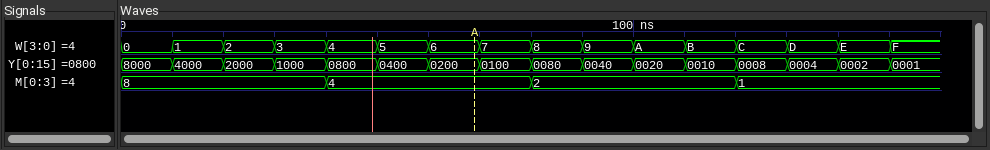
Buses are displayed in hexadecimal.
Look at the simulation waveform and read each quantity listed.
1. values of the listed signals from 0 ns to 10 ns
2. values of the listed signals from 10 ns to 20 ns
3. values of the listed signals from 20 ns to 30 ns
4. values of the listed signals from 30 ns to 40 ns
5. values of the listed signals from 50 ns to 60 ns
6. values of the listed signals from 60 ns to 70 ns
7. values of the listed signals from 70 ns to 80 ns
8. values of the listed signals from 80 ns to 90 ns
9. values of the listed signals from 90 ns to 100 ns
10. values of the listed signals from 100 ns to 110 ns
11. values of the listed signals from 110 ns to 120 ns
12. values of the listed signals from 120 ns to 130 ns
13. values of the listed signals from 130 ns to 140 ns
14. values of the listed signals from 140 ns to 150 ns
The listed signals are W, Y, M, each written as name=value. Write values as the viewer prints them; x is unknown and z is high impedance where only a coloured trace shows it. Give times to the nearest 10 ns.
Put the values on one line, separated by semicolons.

W=0, Y=8000, M=8; W=1, Y=4000, M=8; W=2, Y=2000, M=8; W=3, Y=1000, M=8; W=5, Y=0400, M=4; W=6, Y=0200, M=4; W=7, Y=0100, M=4; W=8, Y=0080, M=2; W=9, Y=0040, M=2; W=A, Y=0020, M=2; W=B, Y=0010, M=2; W=C, Y=0008, M=1; W=D, Y=0004, M=1; W=E, Y=0002, M=1
